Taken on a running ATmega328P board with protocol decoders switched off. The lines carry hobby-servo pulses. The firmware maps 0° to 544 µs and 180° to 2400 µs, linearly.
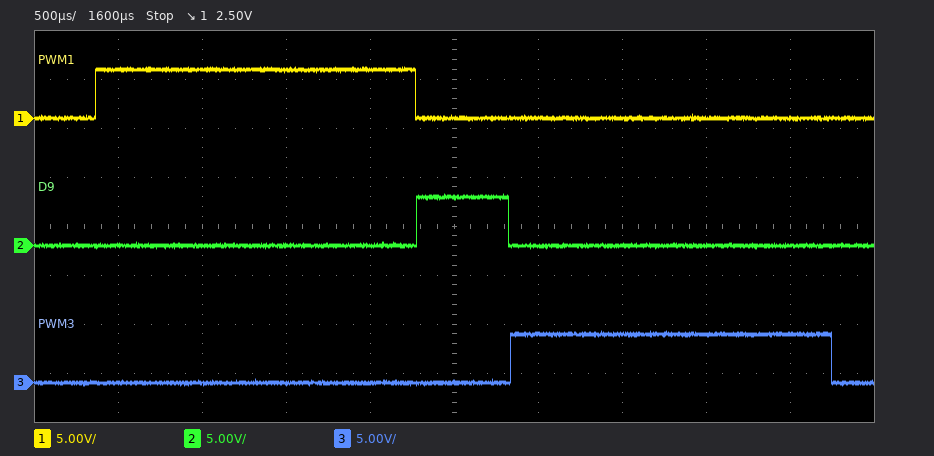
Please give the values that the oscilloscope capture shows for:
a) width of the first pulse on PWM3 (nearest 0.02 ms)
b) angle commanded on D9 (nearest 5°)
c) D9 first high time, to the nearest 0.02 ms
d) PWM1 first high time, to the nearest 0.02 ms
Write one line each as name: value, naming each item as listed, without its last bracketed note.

width of the first pulse on PWM3: 1.92 ms
angle commanded on D9: 0°
D9 first high time, to the nearest 0.02 ms: 0.54 ms
PWM1 first high time, to the nearest 0.02 ms: 1.90 ms
